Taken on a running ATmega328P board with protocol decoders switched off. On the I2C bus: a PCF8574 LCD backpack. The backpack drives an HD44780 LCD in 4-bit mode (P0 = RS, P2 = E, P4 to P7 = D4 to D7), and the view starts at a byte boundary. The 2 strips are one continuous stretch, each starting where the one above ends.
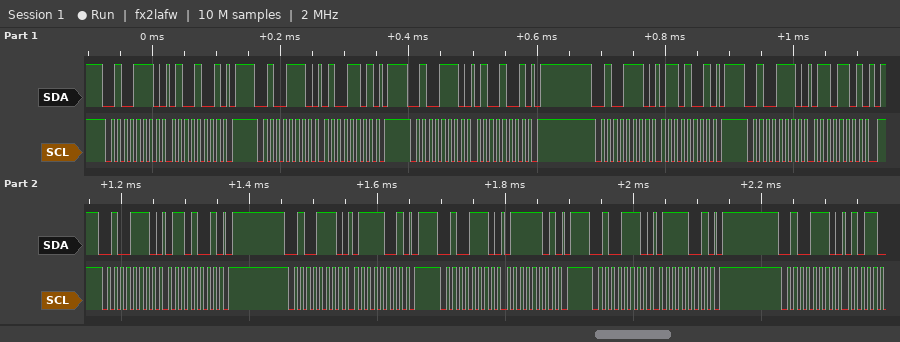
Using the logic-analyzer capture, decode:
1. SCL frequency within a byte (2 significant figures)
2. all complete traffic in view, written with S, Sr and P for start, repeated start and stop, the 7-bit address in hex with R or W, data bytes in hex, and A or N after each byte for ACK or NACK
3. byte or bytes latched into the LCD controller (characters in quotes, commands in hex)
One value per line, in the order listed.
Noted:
100 kHz
S 27W A 49 A P S 27W A 4D A P S 27W A 49 A P S 27W A 69 A P S 27W A 6D A P S 27W A 69 A P S 27W A 79 A P S 27W A 7D A P S 27W A 79 A P S 27W A
'F'
